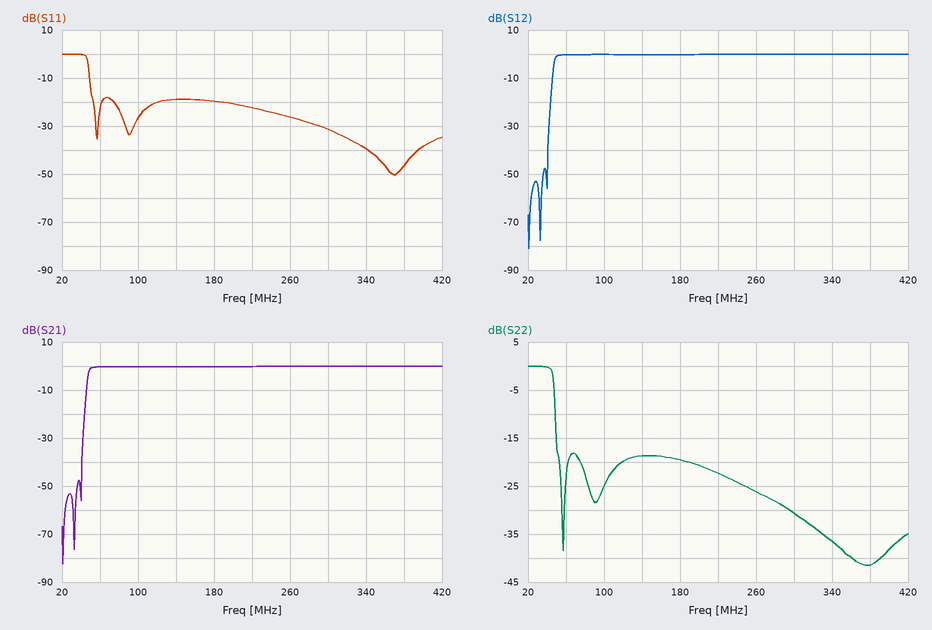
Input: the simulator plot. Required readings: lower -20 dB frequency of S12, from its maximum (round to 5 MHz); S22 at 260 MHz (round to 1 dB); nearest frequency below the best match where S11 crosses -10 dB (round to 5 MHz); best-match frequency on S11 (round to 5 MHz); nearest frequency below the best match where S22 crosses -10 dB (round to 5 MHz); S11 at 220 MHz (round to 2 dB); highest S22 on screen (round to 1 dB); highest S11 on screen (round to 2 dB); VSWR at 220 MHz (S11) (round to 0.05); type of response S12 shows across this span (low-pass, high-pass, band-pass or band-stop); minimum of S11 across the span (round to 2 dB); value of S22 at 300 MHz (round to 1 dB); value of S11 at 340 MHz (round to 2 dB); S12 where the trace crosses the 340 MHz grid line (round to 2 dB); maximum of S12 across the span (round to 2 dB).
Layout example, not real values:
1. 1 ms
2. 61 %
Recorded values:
1. 45 MHz
2. -26 dB
3. 50 MHz
4. 370 MHz
5. 50 MHz
6. -22 dB
7. 0 dB
8. 0 dB
9. 1.15
10. high-pass
11. -50 dB
12. -31 dB
13. -40 dB
14. 0 dB
15. 0 dB
